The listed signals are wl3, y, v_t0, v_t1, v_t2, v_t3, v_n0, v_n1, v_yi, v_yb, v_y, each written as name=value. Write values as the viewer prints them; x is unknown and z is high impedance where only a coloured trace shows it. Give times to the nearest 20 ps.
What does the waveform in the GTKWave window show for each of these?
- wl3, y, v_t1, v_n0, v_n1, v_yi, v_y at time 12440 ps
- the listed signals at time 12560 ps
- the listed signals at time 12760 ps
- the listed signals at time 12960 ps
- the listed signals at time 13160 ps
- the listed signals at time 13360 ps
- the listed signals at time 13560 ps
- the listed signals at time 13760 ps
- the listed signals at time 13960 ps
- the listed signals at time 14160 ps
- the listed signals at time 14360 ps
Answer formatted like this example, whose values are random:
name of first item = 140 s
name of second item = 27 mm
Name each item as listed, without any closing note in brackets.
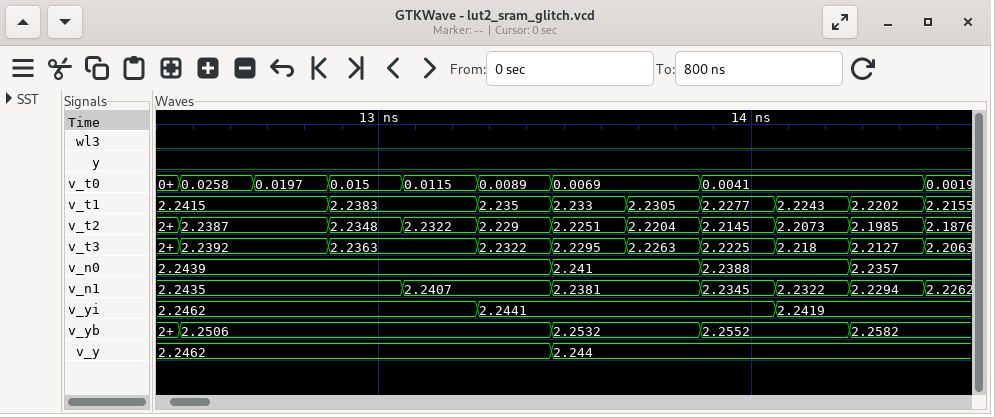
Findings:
wl3, y, v_t1, v_n0, v_n1, v_yi, v_y at time 12440 ps = wl3=0, y=0, v_t1=2.2415, v_n0=2.2439, v_n1=2.2435, v_yi=2.2462, v_y=2.2462
the listed signals at time 12560 ps = wl3=0, y=0, v_t0=0.0258, v_t1=2.2415, v_t2=2.2387, v_t3=2.2392, v_n0=2.2439, v_n1=2.2435, v_yi=2.2462, v_yb=2.2506, v_y=2.2462
the listed signals at time 12760 ps = wl3=0, y=0, v_t0=0.0197, v_t1=2.2415, v_t2=2.2387, v_t3=2.2392, v_n0=2.2439, v_n1=2.2435, v_yi=2.2462, v_yb=2.2506, v_y=2.2462
the listed signals at time 12960 ps = wl3=0, y=0, v_t0=0.015, v_t1=2.2383, v_t2=2.2348, v_t3=2.2363, v_n0=2.2439, v_n1=2.2435, v_yi=2.2462, v_yb=2.2506, v_y=2.2462
the listed signals at time 13160 ps = wl3=0, y=0, v_t0=0.0115, v_t1=2.2383, v_t2=2.2322, v_t3=2.2363, v_n0=2.2439, v_n1=2.2407, v_yi=2.2462, v_yb=2.2506, v_y=2.2462
the listed signals at time 13360 ps = wl3=0, y=0, v_t0=0.0089, v_t1=2.235, v_t2=2.229, v_t3=2.2322, v_n0=2.2439, v_n1=2.2407, v_yi=2.2441, v_yb=2.2506, v_y=2.2462
the listed signals at time 13560 ps = wl3=0, y=0, v_t0=0.0069, v_t1=2.233, v_t2=2.2251, v_t3=2.2295, v_n0=2.241, v_n1=2.2381, v_yi=2.2441, v_yb=2.2532, v_y=2.244
the listed signals at time 13760 ps = wl3=0, y=0, v_t0=0.0069, v_t1=2.2305, v_t2=2.2204, v_t3=2.2263, v_n0=2.241, v_n1=2.2381, v_yi=2.2441, v_yb=2.2532, v_y=2.244
the listed signals at time 13960 ps = wl3=0, y=0, v_t0=0.0041, v_t1=2.2277, v_t2=2.2145, v_t3=2.2225, v_n0=2.2388, v_n1=2.2345, v_yi=2.2441, v_yb=2.2552, v_y=2.244
the listed signals at time 14160 ps = wl3=0, y=0, v_t0=0.0041, v_t1=2.2243, v_t2=2.2073, v_t3=2.218, v_n0=2.2388, v_n1=2.2322, v_yi=2.2419, v_yb=2.2552, v_y=2.244
the listed signals at time 14360 ps = wl3=0, y=0, v_t0=0.0041, v_t1=2.2202, v_t2=2.1985, v_t3=2.2127, v_n0=2.2357, v_n1=2.2294, v_yi=2.2419, v_yb=2.2582, v_y=2.244
